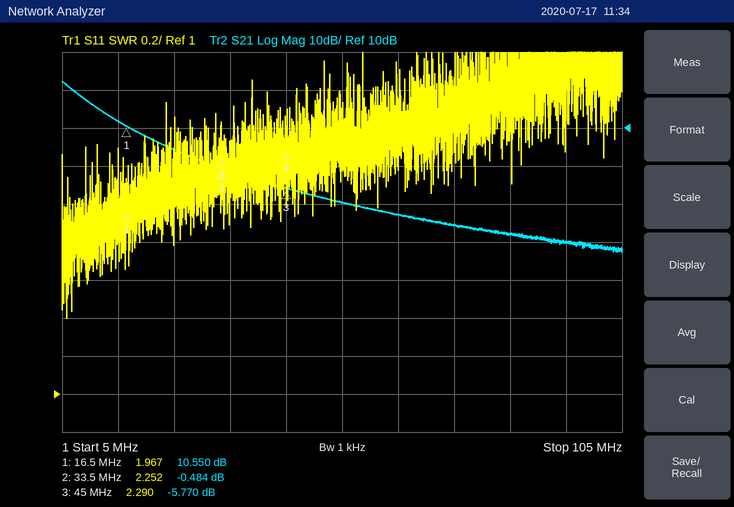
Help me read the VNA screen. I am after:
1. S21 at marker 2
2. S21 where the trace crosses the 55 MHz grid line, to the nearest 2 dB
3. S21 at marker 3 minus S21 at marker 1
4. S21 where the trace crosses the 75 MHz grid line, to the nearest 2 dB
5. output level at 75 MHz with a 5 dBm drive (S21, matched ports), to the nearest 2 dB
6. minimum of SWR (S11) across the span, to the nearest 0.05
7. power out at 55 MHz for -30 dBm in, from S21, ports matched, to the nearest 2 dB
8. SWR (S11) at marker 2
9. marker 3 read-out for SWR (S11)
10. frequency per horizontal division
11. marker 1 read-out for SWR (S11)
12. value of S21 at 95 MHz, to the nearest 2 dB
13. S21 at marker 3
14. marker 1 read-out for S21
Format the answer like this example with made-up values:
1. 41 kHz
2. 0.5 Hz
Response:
1. -0.484 dB
2. -10 dB
3. -16.320 dB
4. -16 dB
5. -10 dBm
6. 1.40
7. -40 dBm
8. 2.252
9. 2.290
10. 10 MHz
11. 1.967
12. -20 dB
13. -5.770 dB
14. 10.550 dB
